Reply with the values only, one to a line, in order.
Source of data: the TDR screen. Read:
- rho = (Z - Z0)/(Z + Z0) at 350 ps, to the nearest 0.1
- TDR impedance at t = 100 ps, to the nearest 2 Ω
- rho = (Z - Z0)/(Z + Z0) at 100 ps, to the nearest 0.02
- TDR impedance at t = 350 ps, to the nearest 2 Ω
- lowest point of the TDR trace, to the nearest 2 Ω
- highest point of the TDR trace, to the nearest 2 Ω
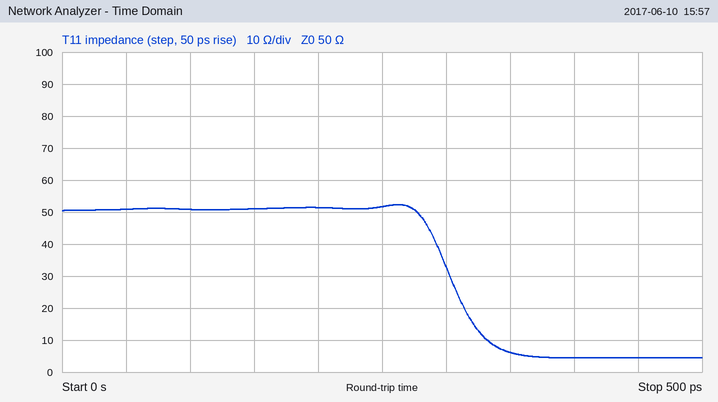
-0.8
50 Ω
0.00
6 Ω
4 Ω
52 Ω
